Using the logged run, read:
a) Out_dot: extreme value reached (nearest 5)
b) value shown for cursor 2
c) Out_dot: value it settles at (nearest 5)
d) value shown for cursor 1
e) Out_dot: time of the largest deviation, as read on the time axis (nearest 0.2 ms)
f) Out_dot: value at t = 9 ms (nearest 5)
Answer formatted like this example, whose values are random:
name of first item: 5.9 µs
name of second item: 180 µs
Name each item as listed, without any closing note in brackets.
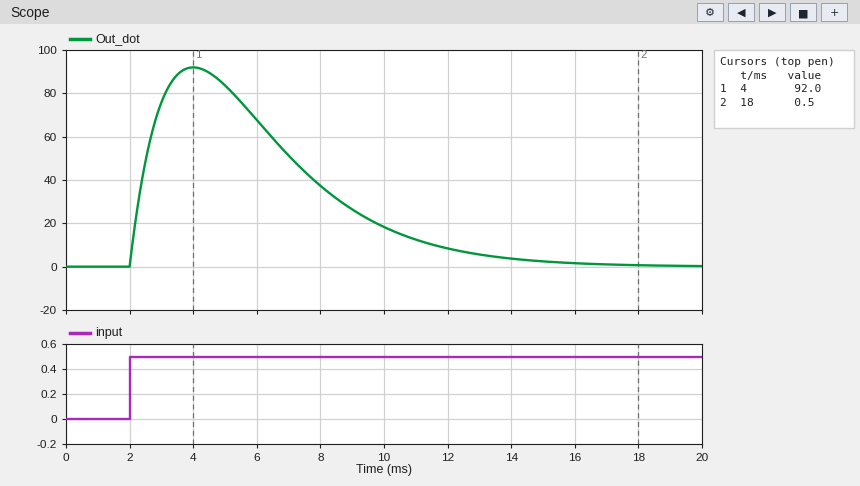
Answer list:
Out_dot: extreme value reached: 90
value shown for cursor 2: 0.5
Out_dot: value it settles at: 0
value shown for cursor 1: 92.0
Out_dot: time of the largest deviation, as read on the time axis: 4.0 ms
Out_dot: value at t = 9 ms: 25
